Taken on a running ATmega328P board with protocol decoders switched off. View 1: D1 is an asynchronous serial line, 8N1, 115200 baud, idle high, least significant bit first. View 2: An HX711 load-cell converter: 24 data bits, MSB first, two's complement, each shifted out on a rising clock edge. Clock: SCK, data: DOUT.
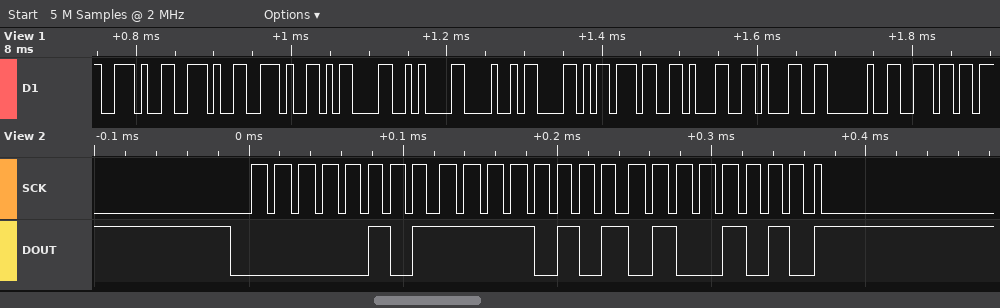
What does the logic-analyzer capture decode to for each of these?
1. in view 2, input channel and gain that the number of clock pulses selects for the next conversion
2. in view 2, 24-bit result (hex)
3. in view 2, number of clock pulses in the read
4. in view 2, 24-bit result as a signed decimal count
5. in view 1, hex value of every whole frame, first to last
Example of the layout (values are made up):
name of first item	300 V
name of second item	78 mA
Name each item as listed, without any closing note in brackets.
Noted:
in view 2, input channel and gain that the number of clock pulses selects for the next conversion	channel A, gain 128
in view 2, 24-bit result	0x05F54A
in view 2, number of clock pulses in the read	25
in view 2, 24-bit result as a signed decimal count	390474
in view 1, hex value of every whole frame, first to last	2E 2E 2E 0D 0A 48 58 37 31 31 20 6E
